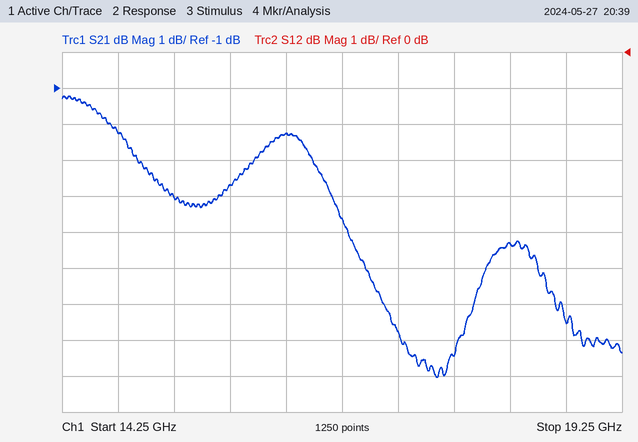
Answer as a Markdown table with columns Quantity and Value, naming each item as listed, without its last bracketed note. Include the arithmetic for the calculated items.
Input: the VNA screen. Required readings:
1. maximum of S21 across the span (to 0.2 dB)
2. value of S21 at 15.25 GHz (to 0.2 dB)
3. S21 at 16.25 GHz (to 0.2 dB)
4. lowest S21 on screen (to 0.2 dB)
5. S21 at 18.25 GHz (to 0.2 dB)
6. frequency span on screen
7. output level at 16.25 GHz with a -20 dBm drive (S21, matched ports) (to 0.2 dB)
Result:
| Quantity | Value |
|---|---|
| maximum of S21 across the span | -1.2 dB |
| value of S21 at 15.25 GHz | -4.0 dB |
| S21 at 16.25 GHz | -2.2 dB |
| lowest S21 on screen | -9.0 dB |
| S21 at 18.25 GHz | -5.4 dB |
| frequency span on screen | 5 GHz |
| output level at 16.25 GHz with a -20 dBm drive (S21, matched ports) | -20 dBm + (-2.2 dB) = -22.2 dBm |
